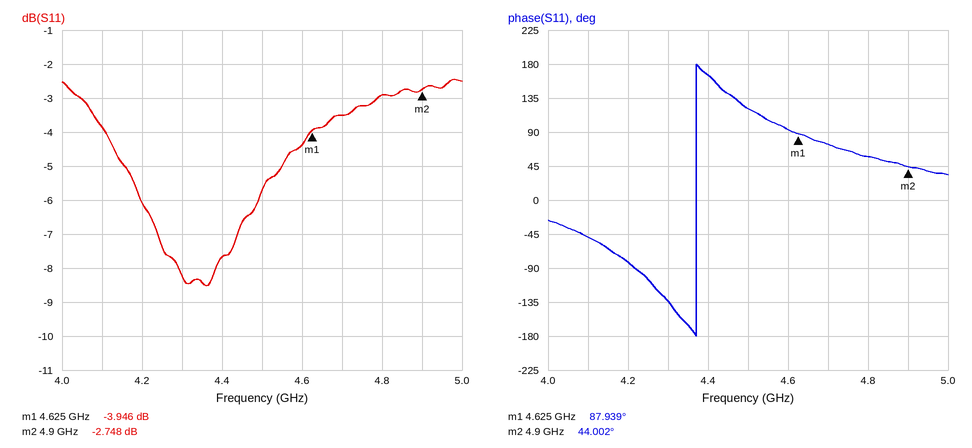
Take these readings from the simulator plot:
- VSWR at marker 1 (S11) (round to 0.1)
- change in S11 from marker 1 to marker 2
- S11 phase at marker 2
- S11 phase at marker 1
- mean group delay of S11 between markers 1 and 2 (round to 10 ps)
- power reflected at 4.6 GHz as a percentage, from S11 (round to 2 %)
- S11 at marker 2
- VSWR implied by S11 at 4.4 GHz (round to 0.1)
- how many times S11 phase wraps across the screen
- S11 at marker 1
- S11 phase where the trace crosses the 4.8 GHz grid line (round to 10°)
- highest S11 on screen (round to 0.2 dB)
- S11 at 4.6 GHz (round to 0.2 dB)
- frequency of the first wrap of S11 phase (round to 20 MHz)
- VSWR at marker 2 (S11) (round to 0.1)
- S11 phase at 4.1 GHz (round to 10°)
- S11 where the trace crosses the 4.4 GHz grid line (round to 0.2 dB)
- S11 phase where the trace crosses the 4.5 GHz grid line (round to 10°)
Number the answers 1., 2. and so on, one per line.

1. 4.5
2. 1.198 dB
3. 44.002°
4. 87.939°
5. 440 ps
6. 36 %
7. -2.748 dB
8. 2.4
9. 1
10. -3.946 dB
11. 60°
12. -2.4 dB
13. -4.4 dB
14. 4.38 GHz
15. 6.4
16. -50°
17. -7.6 dB
18. 120°
